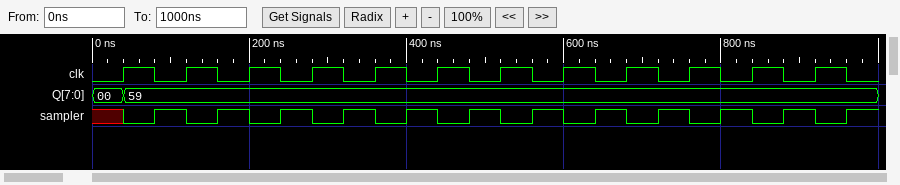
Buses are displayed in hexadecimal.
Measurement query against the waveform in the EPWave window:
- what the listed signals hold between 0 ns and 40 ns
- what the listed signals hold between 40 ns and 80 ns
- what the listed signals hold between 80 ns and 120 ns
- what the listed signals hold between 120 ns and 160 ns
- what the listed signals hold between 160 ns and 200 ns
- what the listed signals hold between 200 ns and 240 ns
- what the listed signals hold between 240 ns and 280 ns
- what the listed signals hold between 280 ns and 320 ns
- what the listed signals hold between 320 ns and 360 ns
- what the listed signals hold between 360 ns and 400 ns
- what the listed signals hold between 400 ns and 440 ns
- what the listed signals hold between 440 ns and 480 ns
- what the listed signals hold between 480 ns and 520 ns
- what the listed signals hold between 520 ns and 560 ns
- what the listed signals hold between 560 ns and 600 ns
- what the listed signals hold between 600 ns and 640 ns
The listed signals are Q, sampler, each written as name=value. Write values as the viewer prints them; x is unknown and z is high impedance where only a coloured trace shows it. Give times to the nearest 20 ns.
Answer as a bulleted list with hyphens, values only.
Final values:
- Q=00, sampler=x
- Q=59, sampler=0
- Q=59, sampler=1
- Q=59, sampler=0
- Q=59, sampler=1
- Q=59, sampler=0
- Q=59, sampler=1
- Q=59, sampler=0
- Q=59, sampler=1
- Q=59, sampler=0
- Q=59, sampler=1
- Q=59, sampler=0
- Q=59, sampler=1
- Q=59, sampler=0
- Q=59, sampler=1
- Q=59, sampler=0
